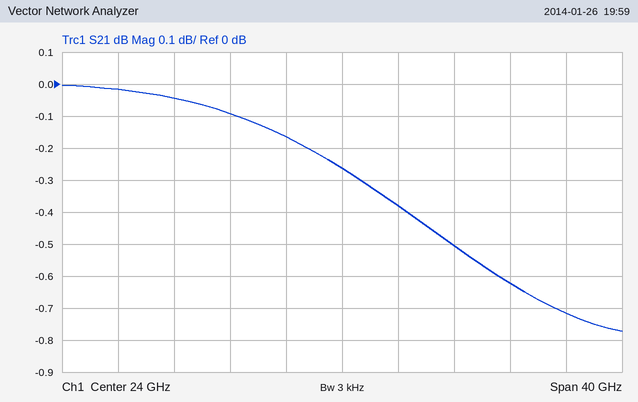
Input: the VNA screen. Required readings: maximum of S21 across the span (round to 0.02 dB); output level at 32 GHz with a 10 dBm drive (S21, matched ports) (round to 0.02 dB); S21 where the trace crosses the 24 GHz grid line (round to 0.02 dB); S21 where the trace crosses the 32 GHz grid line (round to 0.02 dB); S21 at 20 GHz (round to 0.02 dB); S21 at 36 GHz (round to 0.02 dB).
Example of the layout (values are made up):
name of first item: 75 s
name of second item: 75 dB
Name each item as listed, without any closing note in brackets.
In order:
maximum of S21 across the span: 0.00 dB
output level at 32 GHz with a 10 dBm drive (S21, matched ports): 9.50 dBm
S21 where the trace crosses the 24 GHz grid line: -0.26 dB
S21 where the trace crosses the 32 GHz grid line: -0.50 dB
S21 at 20 GHz: -0.16 dB
S21 at 36 GHz: -0.62 dB
